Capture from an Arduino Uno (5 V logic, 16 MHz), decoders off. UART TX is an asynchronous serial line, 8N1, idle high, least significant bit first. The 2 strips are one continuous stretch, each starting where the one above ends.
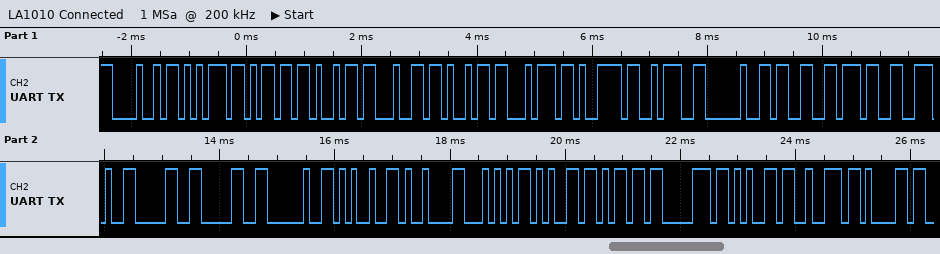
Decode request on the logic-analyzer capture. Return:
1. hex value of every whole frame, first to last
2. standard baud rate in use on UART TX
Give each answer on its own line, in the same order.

48 75 6D 69 64 69 74 79 3A 20 33 37 2E 30 30 20 25 09 54 65 6D 70 65 72 61
9600 baud
